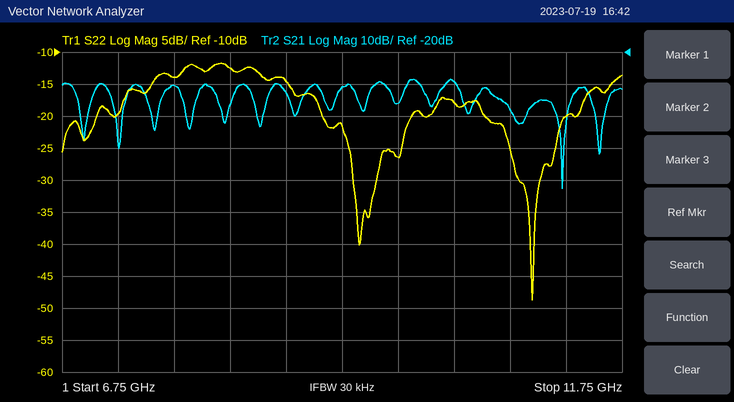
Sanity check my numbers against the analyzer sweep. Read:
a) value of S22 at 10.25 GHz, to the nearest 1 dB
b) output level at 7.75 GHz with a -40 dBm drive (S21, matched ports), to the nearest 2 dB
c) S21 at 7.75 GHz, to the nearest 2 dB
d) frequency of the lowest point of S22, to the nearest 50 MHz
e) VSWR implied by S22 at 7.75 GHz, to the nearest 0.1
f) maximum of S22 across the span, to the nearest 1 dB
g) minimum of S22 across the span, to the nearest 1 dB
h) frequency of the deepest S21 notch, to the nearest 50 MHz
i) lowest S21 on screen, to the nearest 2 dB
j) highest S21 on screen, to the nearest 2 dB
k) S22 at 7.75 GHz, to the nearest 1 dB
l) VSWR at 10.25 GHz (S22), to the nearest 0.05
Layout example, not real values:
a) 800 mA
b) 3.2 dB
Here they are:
a) -18 dB
b) -70 dBm
c) -30 dB
d) 10.95 GHz
e) 1.5
f) -12 dB
g) -49 dB
h) 11.20 GHz
i) -62 dB
j) -28 dB
k) -14 dB
l) 1.30
